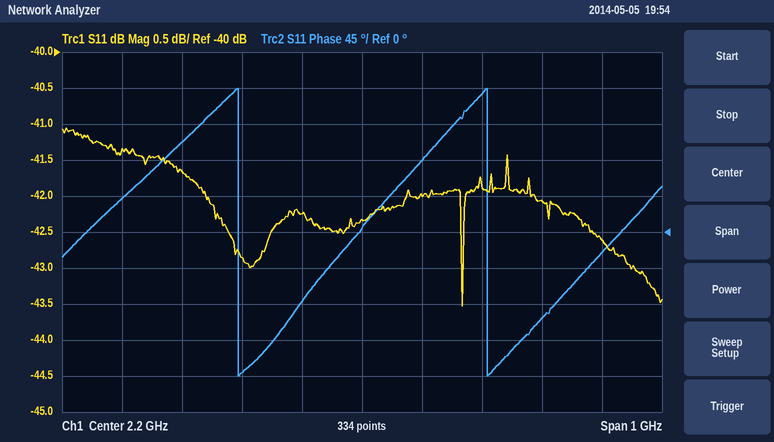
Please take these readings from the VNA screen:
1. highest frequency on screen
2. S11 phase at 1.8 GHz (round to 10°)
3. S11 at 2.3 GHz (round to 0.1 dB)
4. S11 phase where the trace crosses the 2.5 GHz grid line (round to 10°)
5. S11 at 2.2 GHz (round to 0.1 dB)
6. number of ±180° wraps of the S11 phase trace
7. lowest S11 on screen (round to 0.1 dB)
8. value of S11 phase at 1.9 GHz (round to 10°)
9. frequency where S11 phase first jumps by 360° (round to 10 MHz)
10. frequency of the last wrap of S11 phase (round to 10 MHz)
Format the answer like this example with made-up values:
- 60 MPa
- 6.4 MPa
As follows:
- 2.7 GHz
- 40°
- -42.0 dB
- -110°
- -42.3 dB
- 2
- -43.5 dB
- 110°
- 1.99 GHz
- 2.41 GHz
